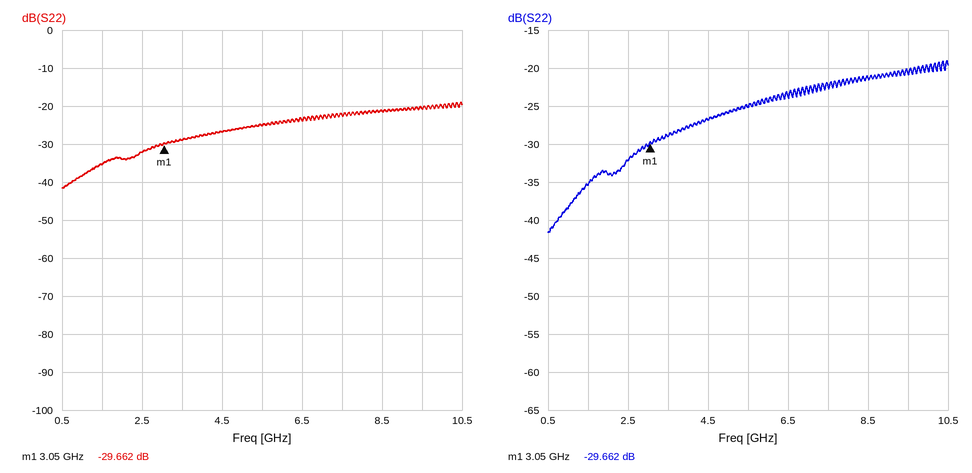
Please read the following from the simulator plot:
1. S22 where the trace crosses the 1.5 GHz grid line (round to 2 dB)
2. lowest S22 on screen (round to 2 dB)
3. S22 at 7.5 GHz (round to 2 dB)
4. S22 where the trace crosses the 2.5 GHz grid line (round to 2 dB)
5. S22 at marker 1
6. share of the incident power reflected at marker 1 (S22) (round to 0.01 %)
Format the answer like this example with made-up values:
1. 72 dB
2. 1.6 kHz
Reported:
1. -36 dB
2. -42 dB
3. -22 dB
4. -32 dB
5. -29.662 dB
6. 0.11 %
